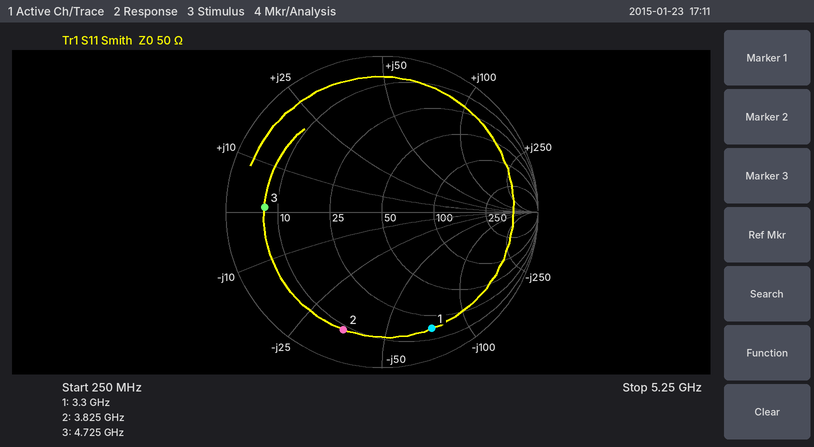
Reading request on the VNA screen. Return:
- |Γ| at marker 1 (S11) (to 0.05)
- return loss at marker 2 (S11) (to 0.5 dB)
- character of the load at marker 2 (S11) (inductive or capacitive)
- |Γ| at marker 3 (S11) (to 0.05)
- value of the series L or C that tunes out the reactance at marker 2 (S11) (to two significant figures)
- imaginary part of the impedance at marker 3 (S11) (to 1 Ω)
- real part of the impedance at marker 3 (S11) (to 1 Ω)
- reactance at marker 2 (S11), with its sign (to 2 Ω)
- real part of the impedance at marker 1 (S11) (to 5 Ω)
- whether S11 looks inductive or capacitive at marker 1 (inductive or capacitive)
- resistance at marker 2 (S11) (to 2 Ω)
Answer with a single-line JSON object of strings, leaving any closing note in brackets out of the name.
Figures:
{"|Γ| at marker 1 (S11)": "0.80", "return loss at marker 2 (S11)": "2.0 dB", "character of the load at marker 2 (S11)": "capacitive", "|Γ| at marker 3 (S11)": "0.75", "value of the series L or C that tunes out the reactance at marker 2 (S11)": "1.5 nH", "imaginary part of the impedance at marker 3 (S11)": "+1 Ω", "real part of the impedance at marker 3 (S11)": "7 Ω", "reactance at marker 2 (S11), with its sign": "-36 Ω", "real part of the impedance at marker 1 (S11)": "15 Ω", "whether S11 looks inductive or capacitive at marker 1": "capacitive", "resistance at marker 2 (S11)": "8 Ω"}
